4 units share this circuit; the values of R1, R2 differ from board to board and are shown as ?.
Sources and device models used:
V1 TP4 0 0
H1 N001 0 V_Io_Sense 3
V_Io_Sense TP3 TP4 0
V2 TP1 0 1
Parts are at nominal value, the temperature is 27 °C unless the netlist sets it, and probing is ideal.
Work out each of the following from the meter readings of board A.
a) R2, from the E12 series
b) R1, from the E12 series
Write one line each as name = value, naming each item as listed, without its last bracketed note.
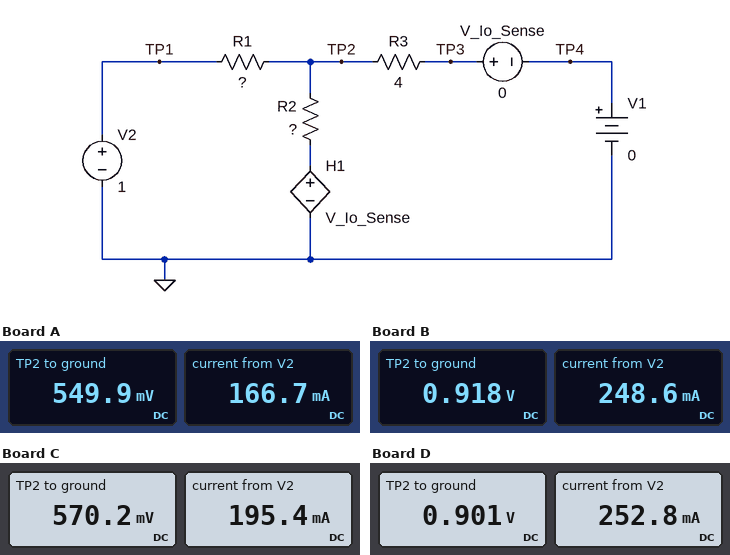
R2, from the E12 series = 4.7 Ω
R1, from the E12 series = 2.7 Ω
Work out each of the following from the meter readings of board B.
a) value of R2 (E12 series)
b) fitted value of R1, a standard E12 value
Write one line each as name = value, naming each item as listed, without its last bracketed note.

value of R2 = 12 Ω
fitted value of R1, a standard E12 value = 0.33 Ω
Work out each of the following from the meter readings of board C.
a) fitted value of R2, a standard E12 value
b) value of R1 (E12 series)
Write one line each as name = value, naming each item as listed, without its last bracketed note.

fitted value of R2, a standard E12 value = 2.7 Ω
value of R1 = 2.2 Ω
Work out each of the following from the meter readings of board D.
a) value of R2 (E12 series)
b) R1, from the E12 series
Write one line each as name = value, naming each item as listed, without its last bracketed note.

value of R2 = 8.2 Ω
R1, from the E12 series = 0.39 Ω
